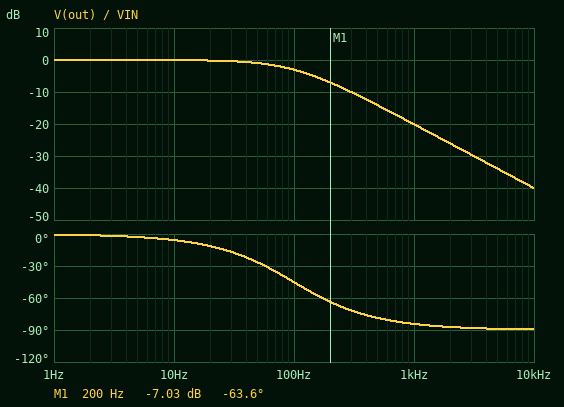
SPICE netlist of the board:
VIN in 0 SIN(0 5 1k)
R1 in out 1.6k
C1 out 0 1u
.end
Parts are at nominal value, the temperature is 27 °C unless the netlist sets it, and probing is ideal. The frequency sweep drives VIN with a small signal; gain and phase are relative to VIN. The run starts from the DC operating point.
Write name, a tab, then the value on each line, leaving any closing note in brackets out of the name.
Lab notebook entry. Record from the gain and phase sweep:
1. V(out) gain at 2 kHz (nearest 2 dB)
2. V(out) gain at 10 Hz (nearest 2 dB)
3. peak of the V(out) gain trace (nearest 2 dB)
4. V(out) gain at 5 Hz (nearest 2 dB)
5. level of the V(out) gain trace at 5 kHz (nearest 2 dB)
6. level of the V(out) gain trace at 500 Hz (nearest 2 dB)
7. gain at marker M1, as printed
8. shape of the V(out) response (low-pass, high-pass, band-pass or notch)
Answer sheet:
V(out) gain at 2 kHz	-26 dB
V(out) gain at 10 Hz	0 dB
peak of the V(out) gain trace	0 dB
V(out) gain at 5 Hz	0 dB
level of the V(out) gain trace at 5 kHz	-34 dB
level of the V(out) gain trace at 500 Hz	-14 dB
gain at marker M1, as printed	-7.03 dB
shape of the V(out) response	low-pass
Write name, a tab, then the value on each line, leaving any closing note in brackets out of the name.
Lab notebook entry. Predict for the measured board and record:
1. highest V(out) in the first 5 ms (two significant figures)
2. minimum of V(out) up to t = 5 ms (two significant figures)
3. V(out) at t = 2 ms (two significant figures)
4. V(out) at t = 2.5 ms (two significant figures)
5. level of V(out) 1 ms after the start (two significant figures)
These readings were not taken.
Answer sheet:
highest V(out) in the first 5 ms	860 mV
minimum of V(out) up to t = 5 ms	-470 mV
V(out) at t = 2 ms	-350 mV
V(out) at t = 2.5 ms	600 mV
level of V(out) 1 ms after the start	-230 mV
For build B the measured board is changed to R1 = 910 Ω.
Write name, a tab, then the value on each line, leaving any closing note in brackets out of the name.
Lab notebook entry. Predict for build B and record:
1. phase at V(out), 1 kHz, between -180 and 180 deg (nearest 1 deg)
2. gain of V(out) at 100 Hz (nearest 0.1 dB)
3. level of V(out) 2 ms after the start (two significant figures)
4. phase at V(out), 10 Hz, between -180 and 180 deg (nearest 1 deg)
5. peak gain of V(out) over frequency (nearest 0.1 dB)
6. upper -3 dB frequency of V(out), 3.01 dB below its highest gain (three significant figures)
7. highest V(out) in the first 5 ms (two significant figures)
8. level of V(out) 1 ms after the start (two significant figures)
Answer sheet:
phase at V(out), 1 kHz, between -180 and 180 deg	-80 deg
gain of V(out) at 100 Hz	-1.2 dB
level of V(out) 2 ms after the start	-750 mV
phase at V(out), 10 Hz, between -180 and 180 deg	-3 deg
peak gain of V(out) over frequency	0 dB
upper -3 dB frequency of V(out), 3.01 dB below its highest gain	175 Hz
highest V(out) in the first 5 ms	1.4 V
level of V(out) 1 ms after the start	-570 mV
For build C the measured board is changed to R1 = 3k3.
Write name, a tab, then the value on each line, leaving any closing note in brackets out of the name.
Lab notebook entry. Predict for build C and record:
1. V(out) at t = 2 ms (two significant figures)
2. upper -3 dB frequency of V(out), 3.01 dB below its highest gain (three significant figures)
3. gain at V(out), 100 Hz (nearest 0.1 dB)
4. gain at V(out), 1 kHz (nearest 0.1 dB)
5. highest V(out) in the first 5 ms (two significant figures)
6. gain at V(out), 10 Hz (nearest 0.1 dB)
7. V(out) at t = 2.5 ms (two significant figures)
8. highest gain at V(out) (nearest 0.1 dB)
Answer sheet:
V(out) at t = 2 ms	-110 mV
upper -3 dB frequency of V(out), 3.01 dB below its highest gain	48.2 Hz
gain at V(out), 100 Hz	-7.2 dB
gain at V(out), 1 kHz	-26.3 dB
highest V(out) in the first 5 ms	450 mV
gain at V(out), 10 Hz	-0.2 dB
V(out) at t = 2.5 ms	350 mV
highest gain at V(out)	0 dB
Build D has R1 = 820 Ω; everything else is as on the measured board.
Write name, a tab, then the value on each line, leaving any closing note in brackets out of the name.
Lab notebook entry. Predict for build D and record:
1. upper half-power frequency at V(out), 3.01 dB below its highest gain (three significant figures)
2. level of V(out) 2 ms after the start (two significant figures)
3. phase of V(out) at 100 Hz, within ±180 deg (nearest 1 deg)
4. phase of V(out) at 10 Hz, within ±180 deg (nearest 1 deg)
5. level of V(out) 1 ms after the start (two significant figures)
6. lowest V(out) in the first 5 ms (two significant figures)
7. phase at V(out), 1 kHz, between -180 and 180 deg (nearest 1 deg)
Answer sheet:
upper half-power frequency at V(out), 3.01 dB below its highest gain	194 Hz
level of V(out) 2 ms after the start	-850 mV
phase of V(out) at 100 Hz, within ±180 deg	-27 deg
phase of V(out) at 10 Hz, within ±180 deg	-3 deg
level of V(out) 1 ms after the start	-660 mV
lowest V(out) in the first 5 ms	-950 mV
phase at V(out), 1 kHz, between -180 and 180 deg	-79 deg
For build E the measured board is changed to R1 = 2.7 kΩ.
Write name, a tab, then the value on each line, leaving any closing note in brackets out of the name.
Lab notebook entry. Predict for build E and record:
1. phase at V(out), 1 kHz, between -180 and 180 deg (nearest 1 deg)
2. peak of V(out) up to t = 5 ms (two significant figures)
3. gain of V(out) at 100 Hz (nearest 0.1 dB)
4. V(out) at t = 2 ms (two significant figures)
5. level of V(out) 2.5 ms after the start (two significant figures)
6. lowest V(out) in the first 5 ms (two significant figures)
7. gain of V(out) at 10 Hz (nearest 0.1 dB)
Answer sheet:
phase at V(out), 1 kHz, between -180 and 180 deg	-87 deg
peak of V(out) up to t = 5 ms	540 mV
gain of V(out) at 100 Hz	-5.9 dB
V(out) at t = 2 ms	-150 mV
level of V(out) 2.5 ms after the start	410 mV
lowest V(out) in the first 5 ms	-250 mV
gain of V(out) at 10 Hz	-0.1 dB
